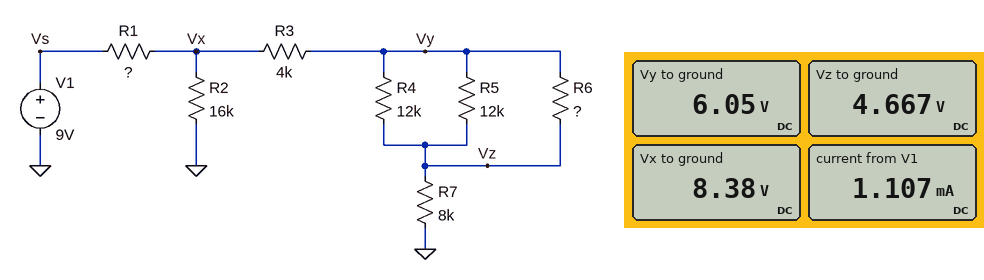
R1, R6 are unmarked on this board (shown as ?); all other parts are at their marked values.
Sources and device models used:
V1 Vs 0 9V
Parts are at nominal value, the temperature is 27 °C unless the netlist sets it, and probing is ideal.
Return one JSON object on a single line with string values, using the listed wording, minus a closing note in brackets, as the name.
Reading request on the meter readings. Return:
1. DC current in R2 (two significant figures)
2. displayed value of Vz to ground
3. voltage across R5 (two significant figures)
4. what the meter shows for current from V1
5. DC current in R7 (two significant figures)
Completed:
{"DC current in R2": "520 µA", "displayed value of Vz to ground": "4.667 V", "voltage across R5": "1.4 V", "what the meter shows for current from V1": "1.107 mA", "DC current in R7": "580 µA"}
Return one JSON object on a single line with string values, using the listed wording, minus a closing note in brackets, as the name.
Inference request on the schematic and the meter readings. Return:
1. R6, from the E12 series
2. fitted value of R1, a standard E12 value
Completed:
{"R6, from the E12 series": "3.9 kΩ", "fitted value of R1, a standard E12 value": "560 Ω"}
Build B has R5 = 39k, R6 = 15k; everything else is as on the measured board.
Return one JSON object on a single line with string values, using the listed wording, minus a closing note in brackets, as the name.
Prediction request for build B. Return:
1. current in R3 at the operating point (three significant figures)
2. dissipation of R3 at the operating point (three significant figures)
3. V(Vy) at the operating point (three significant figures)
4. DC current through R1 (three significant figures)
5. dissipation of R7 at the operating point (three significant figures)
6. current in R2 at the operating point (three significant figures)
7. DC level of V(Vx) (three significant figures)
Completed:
{"current in R3 at the operating point": "477 µA", "dissipation of R3 at the operating point": "910 µW", "V(Vy) at the operating point": "6.53 V", "DC current through R1": "1.00 mA", "dissipation of R7 at the operating point": "1.82 mW", "current in R2 at the operating point": "527 µA", "DC level of V(Vx)": "8.44 V"}
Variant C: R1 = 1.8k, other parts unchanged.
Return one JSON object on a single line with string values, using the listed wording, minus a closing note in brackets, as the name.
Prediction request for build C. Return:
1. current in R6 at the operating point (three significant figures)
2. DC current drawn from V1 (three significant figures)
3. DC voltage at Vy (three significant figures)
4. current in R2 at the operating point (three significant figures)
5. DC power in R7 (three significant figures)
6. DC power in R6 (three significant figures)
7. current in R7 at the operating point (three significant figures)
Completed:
{"current in R6 at the operating point": "307 µA", "DC current drawn from V1": "961 µA", "DC voltage at Vy": "5.25 V", "current in R2 at the operating point": "454 µA", "DC power in R7": "2.05 mW", "DC power in R6": "367 µW", "current in R7 at the operating point": "506 µA"}
